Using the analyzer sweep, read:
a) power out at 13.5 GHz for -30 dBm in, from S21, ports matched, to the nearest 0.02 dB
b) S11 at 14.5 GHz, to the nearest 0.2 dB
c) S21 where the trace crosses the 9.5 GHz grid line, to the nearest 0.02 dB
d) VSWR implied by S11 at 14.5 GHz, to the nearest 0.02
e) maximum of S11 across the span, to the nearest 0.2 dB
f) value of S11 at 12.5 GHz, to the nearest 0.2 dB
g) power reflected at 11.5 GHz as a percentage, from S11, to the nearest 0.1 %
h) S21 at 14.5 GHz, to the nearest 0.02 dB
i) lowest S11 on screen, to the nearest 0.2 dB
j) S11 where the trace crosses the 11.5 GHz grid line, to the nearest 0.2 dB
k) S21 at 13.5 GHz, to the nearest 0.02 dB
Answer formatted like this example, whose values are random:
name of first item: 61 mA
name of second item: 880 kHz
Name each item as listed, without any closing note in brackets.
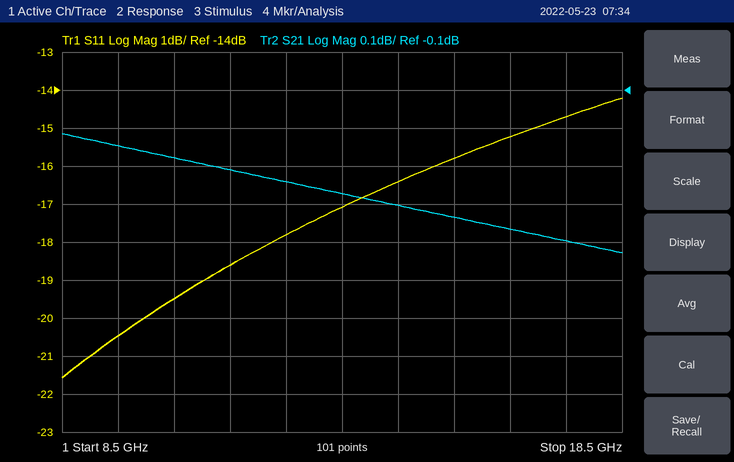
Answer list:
power out at 13.5 GHz for -30 dBm in, from S21, ports matched, to the nearest 0.02 dB: -30.38 dBm
S11 at 14.5 GHz, to the nearest 0.2 dB: -16.4 dB
S21 where the trace crosses the 9.5 GHz grid line, to the nearest 0.02 dB: -0.24 dB
VSWR implied by S11 at 14.5 GHz, to the nearest 0.02: 1.36
maximum of S11 across the span, to the nearest 0.2 dB: -14.2 dB
value of S11 at 12.5 GHz, to the nearest 0.2 dB: -17.8 dB
power reflected at 11.5 GHz as a percentage, from S11, to the nearest 0.1 %: 1.4 %
S21 at 14.5 GHz, to the nearest 0.02 dB: -0.40 dB
lowest S11 on screen, to the nearest 0.2 dB: -21.6 dB
S11 where the trace crosses the 11.5 GHz grid line, to the nearest 0.2 dB: -18.6 dB
S21 at 13.5 GHz, to the nearest 0.02 dB: -0.38 dB
